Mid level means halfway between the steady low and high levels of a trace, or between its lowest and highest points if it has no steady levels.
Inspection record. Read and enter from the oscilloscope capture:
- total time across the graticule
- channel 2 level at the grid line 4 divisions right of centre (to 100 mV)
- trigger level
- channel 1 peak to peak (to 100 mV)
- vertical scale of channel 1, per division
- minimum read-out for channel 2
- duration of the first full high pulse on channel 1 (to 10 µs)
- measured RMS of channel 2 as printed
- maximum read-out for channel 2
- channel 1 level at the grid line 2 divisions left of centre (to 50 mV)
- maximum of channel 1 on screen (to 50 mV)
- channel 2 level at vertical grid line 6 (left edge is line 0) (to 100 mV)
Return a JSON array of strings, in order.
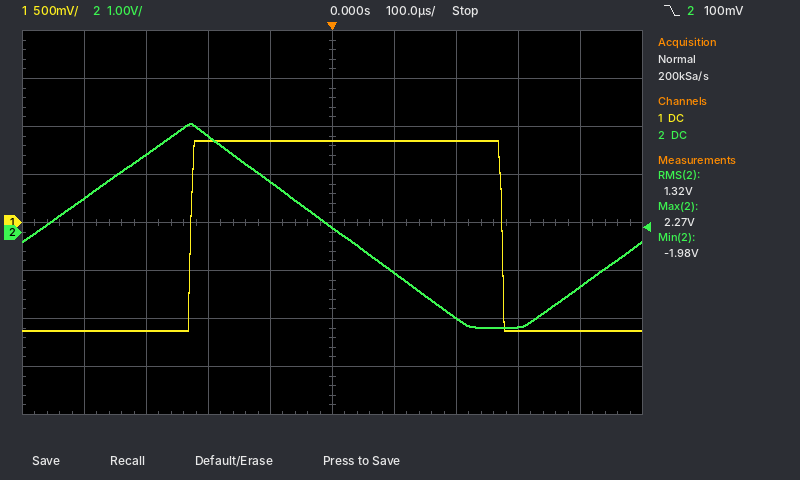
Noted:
["1 ms", "-1.1 V", "100 mV", "2.00 V", "500 mV", "-1.98 V", "500 µs", "1.32 V", "2.27 V", "850 mV", "850 mV", "-800 mV"]
